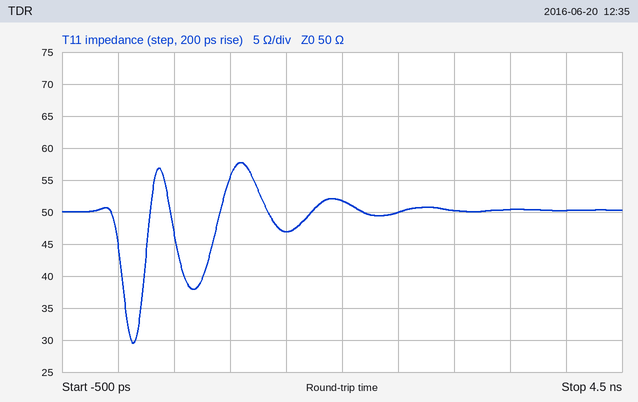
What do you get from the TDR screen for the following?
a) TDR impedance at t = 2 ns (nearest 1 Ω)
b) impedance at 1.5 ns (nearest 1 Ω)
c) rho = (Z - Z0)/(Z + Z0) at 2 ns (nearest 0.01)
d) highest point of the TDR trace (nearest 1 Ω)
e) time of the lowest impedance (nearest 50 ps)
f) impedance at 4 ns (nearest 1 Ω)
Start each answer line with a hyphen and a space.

- 52 Ω
- 47 Ω
- +0.02
- 58 Ω
- 150 ps
- 50 Ω
